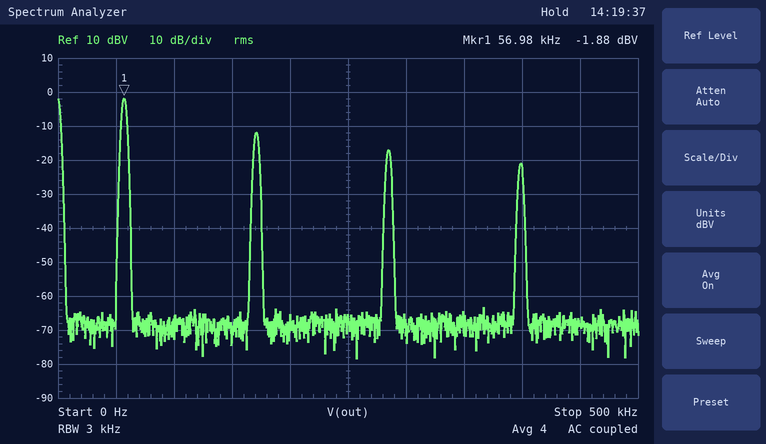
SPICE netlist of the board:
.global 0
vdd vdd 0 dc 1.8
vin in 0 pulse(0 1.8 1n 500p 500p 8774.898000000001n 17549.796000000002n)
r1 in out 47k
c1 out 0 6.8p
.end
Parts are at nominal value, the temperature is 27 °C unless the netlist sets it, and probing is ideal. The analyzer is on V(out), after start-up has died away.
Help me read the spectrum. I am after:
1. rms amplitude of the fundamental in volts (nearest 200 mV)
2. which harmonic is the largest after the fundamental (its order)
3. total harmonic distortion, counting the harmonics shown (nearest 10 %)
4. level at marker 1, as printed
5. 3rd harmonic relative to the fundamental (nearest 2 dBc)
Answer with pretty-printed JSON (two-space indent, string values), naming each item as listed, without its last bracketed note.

{
  "rms amplitude of the fundamental in volts": "800 mV",
  "which harmonic is the largest after the fundamental": "3",
  "total harmonic distortion, counting the harmonics shown": "40 %",
  "level at marker 1, as printed": "-1.88 dBV",
  "3rd harmonic relative to the fundamental": "-10 dBc"
}
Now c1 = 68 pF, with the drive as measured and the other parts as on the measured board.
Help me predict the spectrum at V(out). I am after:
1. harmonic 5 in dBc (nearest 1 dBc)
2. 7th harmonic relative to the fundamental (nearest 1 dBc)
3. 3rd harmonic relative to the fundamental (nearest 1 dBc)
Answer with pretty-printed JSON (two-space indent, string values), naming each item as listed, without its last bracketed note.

{
  "harmonic 5 in dBc": "-26 dBc",
  "7th harmonic relative to the fundamental": "-31 dBc",
  "3rd harmonic relative to the fundamental": "-17 dBc"
}
